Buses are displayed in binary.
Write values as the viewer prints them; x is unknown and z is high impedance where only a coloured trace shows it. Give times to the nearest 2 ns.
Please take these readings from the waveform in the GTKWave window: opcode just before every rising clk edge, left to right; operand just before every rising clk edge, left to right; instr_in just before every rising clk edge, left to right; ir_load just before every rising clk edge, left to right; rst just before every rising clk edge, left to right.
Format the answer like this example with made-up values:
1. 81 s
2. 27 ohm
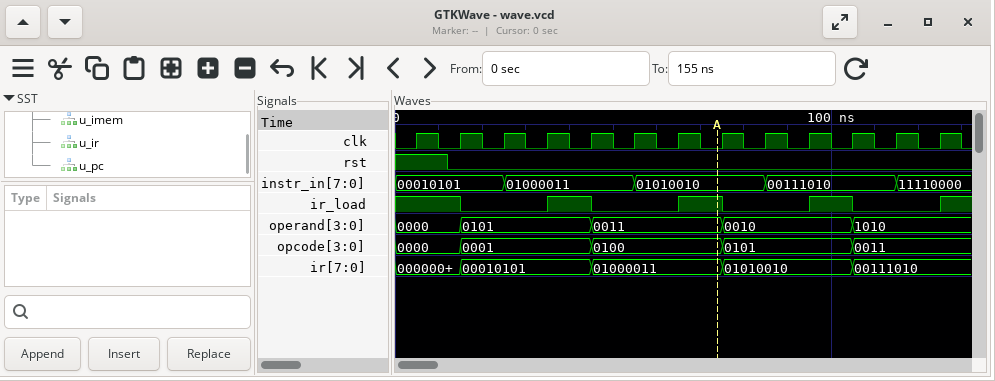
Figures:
1. 0000, 0000, 0001, 0001, 0001, 0100, 0100, 0100, 0101, 0101, 0101, 0011, 0011
2. 0000, 0000, 0101, 0101, 0101, 0011, 0011, 0011, 0010, 0010, 0010, 1010, 1010
3. 00010101, 00010101, 00010101, 01000011, 01000011, 01000011, 01010010, 01010010, 01010010, 00111010, 00111010, 00111010, 11110000
4. 1 1 0 0 1 0 0 1 0 0 1 0 0
5. 1 0 0 0 0 0 0 0 0 0 0 0 0
